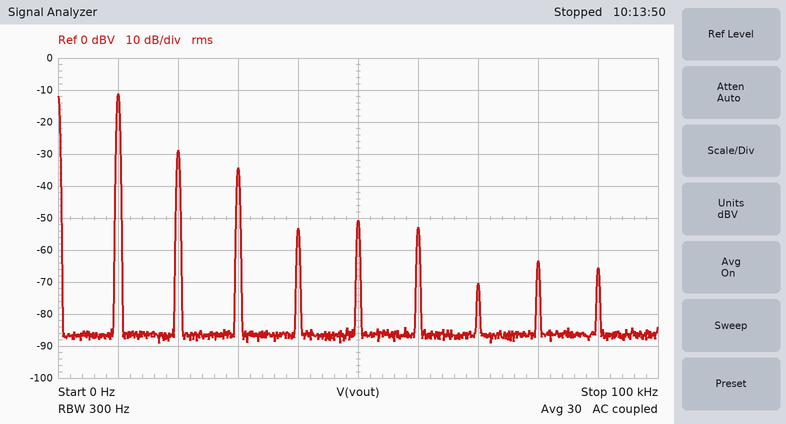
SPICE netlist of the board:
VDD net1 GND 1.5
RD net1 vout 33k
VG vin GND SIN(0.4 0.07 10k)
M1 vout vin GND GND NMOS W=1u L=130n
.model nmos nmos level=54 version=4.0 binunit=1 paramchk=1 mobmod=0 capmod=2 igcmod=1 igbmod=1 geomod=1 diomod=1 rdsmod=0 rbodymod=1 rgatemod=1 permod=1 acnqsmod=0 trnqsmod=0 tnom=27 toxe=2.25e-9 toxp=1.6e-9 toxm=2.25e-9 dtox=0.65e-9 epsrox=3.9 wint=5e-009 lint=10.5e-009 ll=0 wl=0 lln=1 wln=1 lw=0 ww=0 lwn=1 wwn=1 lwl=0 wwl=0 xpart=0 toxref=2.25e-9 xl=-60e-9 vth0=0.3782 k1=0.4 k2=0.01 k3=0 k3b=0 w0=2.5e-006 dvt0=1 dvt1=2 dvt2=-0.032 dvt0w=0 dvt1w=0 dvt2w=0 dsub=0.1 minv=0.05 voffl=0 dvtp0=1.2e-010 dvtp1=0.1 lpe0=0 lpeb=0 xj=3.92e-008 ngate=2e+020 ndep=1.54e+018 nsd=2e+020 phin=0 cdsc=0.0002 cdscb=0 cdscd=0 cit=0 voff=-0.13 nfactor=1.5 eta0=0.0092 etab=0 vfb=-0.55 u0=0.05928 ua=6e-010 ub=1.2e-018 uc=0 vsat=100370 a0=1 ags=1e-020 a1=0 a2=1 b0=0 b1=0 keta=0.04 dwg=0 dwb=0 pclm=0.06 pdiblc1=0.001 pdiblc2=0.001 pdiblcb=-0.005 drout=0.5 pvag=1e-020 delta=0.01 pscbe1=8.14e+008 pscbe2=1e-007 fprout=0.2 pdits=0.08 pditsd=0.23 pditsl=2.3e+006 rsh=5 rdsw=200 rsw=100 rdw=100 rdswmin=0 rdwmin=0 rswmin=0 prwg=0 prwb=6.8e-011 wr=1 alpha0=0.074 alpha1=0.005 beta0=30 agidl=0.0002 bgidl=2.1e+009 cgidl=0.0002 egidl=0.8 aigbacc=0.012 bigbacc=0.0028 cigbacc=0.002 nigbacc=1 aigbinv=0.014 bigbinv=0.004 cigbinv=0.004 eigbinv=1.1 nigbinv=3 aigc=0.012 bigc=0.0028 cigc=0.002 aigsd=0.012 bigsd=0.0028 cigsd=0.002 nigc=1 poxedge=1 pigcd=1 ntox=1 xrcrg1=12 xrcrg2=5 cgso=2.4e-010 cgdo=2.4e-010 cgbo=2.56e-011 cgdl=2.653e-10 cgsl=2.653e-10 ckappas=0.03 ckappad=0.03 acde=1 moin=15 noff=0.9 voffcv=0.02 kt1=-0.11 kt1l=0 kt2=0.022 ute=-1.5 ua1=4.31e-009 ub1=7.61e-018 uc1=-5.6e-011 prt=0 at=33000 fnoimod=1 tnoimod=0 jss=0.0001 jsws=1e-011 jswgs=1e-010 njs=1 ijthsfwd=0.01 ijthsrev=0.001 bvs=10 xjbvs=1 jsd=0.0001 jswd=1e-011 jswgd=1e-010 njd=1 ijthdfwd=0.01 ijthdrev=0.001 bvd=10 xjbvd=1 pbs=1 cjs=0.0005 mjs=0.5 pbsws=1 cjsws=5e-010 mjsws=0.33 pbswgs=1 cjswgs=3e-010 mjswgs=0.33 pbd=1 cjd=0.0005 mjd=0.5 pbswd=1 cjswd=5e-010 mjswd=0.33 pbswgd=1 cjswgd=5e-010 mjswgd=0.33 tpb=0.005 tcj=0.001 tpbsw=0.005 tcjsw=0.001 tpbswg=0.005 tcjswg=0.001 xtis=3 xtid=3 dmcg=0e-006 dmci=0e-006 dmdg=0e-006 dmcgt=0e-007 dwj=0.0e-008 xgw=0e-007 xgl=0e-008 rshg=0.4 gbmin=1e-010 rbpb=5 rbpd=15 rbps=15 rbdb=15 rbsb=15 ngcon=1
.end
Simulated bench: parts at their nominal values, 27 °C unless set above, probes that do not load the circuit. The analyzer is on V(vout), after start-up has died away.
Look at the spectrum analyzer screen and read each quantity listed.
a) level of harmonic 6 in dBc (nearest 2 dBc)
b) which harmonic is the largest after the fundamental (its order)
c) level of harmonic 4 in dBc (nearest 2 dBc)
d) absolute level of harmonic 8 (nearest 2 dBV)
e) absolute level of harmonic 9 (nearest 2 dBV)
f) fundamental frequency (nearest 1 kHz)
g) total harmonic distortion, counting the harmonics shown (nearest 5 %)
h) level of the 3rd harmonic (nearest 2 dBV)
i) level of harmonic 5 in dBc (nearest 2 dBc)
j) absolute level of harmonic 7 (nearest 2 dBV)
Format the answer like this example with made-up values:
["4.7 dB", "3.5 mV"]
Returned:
["-42 dBc", "2", "-42 dBc", "-64 dBV", "-66 dBV", "10 kHz", "15 %", "-34 dBV", "-40 dBc", "-70 dBV"]
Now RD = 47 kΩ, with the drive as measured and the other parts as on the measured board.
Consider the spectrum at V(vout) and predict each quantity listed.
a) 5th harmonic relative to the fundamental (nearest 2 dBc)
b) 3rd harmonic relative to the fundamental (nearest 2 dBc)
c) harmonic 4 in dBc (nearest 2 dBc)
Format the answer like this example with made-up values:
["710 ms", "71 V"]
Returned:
["-36 dBc", "-26 dBc", "-28 dBc"]
